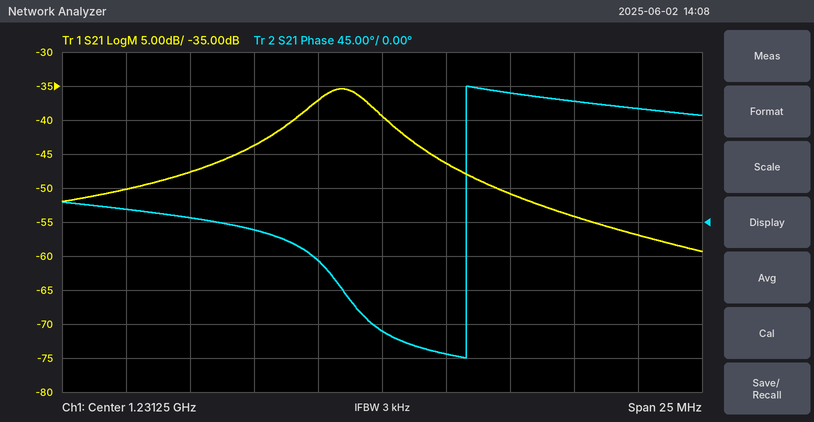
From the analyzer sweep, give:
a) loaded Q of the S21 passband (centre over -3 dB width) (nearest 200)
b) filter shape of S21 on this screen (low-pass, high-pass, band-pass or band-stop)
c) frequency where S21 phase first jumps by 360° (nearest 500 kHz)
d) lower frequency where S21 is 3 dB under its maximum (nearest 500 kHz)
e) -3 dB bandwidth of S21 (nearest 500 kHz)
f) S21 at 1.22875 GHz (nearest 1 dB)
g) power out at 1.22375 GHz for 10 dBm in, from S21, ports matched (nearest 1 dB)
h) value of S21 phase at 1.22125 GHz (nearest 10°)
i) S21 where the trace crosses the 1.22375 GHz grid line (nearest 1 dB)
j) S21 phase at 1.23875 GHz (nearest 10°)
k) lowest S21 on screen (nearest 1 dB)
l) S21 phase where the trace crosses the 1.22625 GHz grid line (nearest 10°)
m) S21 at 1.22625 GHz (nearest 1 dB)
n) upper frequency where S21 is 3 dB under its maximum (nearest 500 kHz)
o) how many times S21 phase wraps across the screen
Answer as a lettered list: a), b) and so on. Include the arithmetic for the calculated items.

a) 1.22975 GHz / 2.5 MHz ≈ 492, so 400 to the nearest 200
b) band-pass
c) 1.2345 GHz
d) 1.2285 GHz
e) 1.2310 GHz − 1.2285 GHz = 2.5 MHz
f) -37 dB
g) 10 dBm + (-48 dB) = -38 dBm
h) 20°
i) -48 dB
j) 160°
k) -59 dB
l) -10°
m) -44 dB
n) 1.2310 GHz
o) 1
